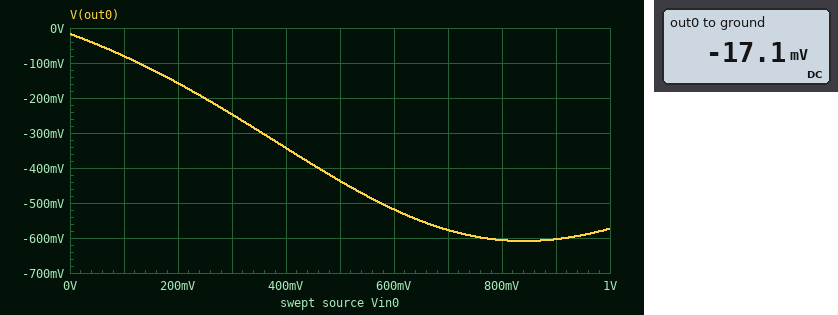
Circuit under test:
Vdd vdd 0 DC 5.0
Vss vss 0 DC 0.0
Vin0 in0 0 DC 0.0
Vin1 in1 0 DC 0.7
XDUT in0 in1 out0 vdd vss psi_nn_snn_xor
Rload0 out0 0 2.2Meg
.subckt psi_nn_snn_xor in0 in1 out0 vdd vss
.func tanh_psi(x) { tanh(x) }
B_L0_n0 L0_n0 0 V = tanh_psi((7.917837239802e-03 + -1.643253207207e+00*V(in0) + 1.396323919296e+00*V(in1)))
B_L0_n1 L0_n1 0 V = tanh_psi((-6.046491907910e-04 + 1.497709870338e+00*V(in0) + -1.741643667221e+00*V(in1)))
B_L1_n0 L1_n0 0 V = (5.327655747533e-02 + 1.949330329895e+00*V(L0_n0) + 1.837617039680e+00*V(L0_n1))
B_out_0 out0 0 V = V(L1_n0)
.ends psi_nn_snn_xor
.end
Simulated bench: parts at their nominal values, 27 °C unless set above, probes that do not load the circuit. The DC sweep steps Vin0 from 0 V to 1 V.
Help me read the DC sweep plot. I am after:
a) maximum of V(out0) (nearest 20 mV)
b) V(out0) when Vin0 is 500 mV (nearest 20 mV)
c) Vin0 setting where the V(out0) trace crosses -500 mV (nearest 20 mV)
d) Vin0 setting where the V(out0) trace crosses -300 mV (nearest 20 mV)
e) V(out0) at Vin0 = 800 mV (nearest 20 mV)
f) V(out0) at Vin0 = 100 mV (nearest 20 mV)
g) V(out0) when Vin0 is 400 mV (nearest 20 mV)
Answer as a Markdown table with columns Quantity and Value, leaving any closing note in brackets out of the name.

| Quantity | Value |
|---|---|
| maximum of V(out0) | -20 mV |
| V(out0) when Vin0 is 500 mV | -440 mV |
| Vin0 setting where the V(out0) trace crosses -500 mV | 580 mV |
| Vin0 setting where the V(out0) trace crosses -300 mV | 360 mV |
| V(out0) at Vin0 = 800 mV | -600 mV |
| V(out0) at Vin0 = 100 mV | -80 mV |
| V(out0) when Vin0 is 400 mV | -340 mV |
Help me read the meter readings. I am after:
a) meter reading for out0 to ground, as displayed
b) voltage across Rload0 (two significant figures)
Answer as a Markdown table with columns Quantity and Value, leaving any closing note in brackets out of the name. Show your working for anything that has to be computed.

| Quantity | Value |
|---|---|
| meter reading for out0 to ground, as displayed | -17.1 mV |
| voltage across Rload0 | 0 V - (-17.1 mV) = 17 mV |
